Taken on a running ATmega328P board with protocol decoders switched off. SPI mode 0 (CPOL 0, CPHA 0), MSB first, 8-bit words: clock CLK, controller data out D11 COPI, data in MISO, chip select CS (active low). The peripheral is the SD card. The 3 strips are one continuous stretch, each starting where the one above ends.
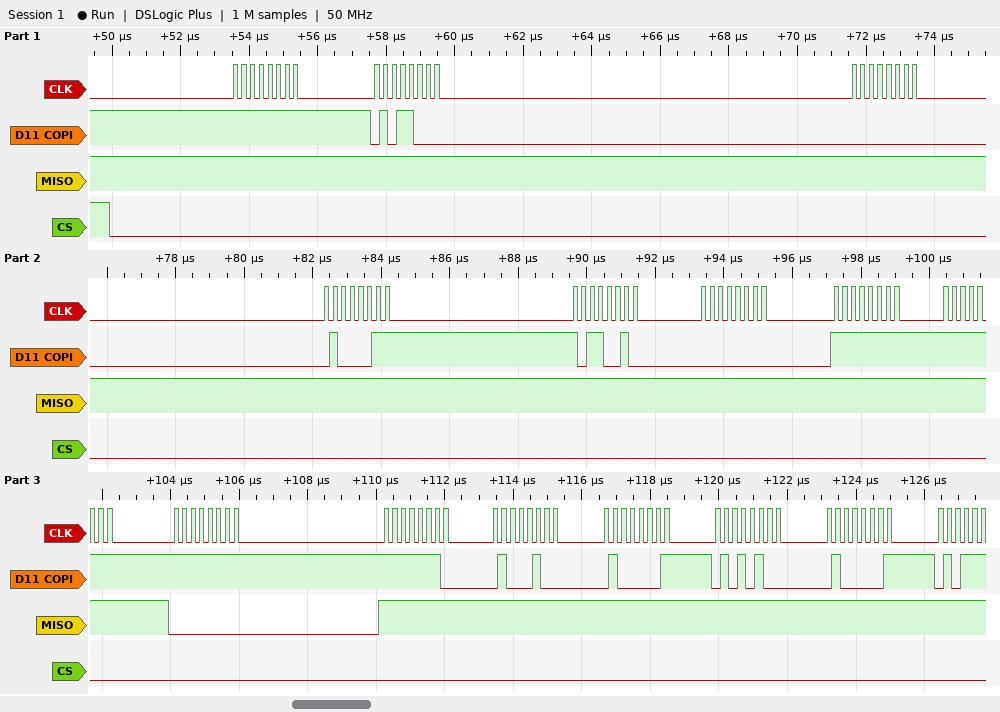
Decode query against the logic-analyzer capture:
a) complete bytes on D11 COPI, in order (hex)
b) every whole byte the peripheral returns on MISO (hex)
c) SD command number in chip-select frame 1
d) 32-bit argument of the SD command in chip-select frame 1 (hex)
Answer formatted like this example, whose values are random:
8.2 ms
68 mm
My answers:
0xFF 0x58 0x00 0x43 0xB2 0x00 0xFF 0xFF 0xFF 0xFE 0x44 0x41 0x54 0x41
0xFF 0xFF 0xFF 0xFF 0xFF 0xFF 0xFF 0xFF 0x00 0xFF 0xFF 0xFF 0xFF 0xFF
CMD24
0x0043B200
